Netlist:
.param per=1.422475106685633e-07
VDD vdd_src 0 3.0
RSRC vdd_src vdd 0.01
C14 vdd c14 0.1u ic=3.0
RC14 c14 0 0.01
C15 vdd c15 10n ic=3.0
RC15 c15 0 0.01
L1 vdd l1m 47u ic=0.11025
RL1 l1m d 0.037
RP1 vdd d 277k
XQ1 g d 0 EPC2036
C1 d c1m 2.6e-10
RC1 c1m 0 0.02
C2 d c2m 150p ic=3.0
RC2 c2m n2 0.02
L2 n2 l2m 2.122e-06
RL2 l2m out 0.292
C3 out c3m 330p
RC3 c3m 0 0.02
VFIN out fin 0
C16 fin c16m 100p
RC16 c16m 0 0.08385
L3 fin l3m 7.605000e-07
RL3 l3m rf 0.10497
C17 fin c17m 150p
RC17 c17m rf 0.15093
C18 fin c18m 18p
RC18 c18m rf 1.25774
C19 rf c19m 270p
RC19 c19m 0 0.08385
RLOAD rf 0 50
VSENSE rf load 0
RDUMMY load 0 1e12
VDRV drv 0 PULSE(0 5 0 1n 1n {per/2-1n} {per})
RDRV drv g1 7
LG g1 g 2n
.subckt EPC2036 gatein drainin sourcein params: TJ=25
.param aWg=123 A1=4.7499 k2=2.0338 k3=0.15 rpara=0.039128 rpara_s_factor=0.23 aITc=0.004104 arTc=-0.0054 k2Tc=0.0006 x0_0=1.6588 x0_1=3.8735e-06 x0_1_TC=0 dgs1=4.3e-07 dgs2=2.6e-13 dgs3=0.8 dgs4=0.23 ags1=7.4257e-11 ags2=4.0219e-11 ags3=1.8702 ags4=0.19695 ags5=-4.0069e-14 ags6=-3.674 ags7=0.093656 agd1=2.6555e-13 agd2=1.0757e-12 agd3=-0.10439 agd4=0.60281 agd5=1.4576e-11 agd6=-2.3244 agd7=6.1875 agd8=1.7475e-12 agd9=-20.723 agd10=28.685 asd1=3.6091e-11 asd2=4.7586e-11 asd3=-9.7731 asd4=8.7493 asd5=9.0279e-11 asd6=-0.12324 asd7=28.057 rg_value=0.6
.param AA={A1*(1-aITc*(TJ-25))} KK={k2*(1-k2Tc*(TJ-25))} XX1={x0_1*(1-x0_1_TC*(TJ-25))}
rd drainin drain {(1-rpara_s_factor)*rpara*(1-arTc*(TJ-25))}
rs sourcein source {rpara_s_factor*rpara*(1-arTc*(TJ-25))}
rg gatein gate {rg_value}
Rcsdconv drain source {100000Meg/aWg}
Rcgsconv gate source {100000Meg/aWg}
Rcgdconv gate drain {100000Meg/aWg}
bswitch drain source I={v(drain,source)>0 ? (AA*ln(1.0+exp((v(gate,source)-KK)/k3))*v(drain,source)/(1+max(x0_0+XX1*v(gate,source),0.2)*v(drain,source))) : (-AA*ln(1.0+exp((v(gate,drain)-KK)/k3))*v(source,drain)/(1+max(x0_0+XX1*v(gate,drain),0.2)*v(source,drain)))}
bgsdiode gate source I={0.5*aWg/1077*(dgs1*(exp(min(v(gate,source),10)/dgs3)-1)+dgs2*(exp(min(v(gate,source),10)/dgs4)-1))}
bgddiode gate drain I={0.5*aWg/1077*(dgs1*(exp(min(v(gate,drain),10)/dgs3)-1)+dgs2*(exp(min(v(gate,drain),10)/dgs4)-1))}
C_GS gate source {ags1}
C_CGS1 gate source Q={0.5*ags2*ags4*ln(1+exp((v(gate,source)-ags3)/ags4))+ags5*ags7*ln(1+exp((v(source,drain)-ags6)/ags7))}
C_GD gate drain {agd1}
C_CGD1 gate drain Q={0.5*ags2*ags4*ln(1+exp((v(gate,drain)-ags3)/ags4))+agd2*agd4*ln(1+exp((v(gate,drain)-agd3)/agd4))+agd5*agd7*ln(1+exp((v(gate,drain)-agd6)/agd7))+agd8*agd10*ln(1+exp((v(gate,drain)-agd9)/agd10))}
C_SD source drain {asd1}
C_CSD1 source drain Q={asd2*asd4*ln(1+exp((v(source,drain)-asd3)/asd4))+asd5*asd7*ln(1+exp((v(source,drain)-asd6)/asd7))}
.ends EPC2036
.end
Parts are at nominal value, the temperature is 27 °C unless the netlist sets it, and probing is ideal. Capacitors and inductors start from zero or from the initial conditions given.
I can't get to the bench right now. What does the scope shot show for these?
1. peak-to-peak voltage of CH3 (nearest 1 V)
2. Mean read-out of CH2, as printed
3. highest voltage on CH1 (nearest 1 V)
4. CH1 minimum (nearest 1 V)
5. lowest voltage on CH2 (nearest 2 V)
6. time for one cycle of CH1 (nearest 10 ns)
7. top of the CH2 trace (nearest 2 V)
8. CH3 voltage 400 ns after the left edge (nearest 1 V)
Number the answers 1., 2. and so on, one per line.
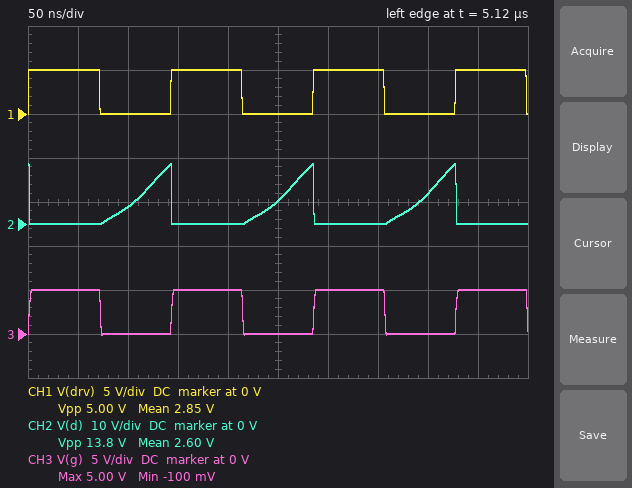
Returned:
1. 5 V
2. 2.60 V
3. 5 V
4. 0 V
5. 0 V
6. 140 ns
7. 14 V
8. 0 V
